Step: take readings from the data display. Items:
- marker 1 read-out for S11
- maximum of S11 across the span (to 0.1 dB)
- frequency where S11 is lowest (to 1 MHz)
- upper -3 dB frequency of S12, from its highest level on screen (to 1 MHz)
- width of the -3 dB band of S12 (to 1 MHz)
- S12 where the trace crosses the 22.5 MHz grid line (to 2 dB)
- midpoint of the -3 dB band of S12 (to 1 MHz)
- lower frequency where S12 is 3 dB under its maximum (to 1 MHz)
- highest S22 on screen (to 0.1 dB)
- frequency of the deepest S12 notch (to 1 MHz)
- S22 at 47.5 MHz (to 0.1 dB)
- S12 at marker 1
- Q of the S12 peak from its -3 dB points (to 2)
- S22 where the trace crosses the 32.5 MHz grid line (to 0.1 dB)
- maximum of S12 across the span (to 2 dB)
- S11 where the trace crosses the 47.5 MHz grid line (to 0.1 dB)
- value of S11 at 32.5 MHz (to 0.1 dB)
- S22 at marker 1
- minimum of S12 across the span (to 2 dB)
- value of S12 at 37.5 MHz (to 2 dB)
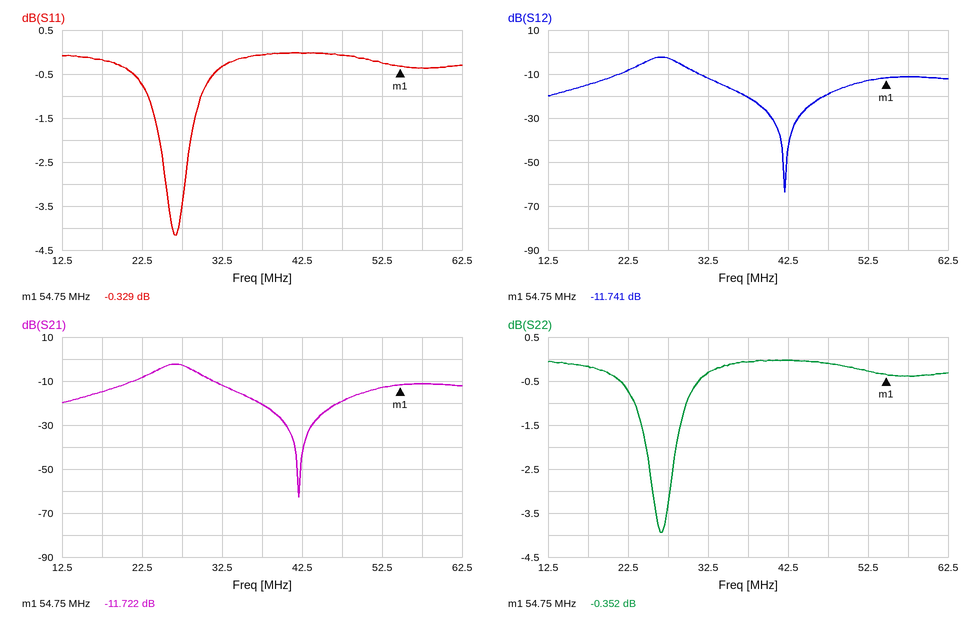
-0.329 dB
0.0 dB
27 MHz
29 MHz
5 MHz
-8 dB
27 MHz
24 MHz
0.0 dB
42 MHz
-0.1 dB
-11.741 dB
6
-0.3 dB
-2 dB
-0.1 dB
-0.3 dB
-0.352 dB
-64 dB
-20 dB
